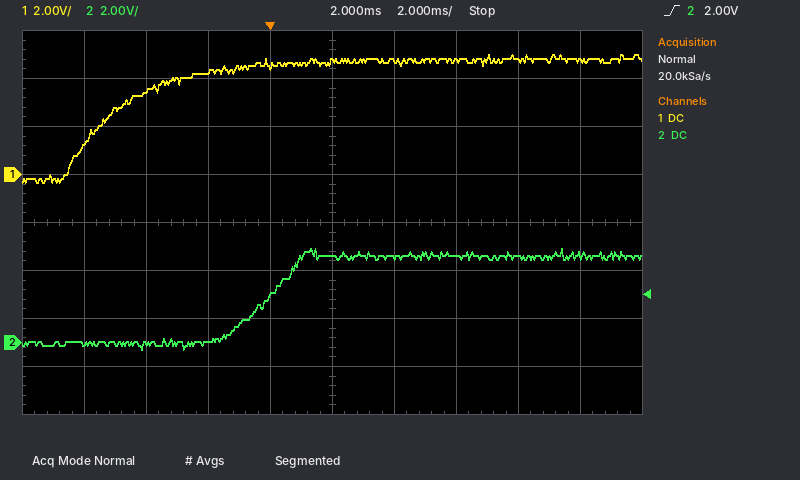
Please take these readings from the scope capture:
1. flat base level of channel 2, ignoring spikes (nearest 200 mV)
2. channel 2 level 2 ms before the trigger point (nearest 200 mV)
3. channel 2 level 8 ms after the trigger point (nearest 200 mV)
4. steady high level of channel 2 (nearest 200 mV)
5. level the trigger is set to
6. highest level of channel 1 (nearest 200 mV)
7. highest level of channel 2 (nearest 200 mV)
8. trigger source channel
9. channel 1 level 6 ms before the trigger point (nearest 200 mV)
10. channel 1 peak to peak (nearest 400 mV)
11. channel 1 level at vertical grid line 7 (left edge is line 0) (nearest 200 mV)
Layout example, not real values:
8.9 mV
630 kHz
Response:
0.0 V
0.0 V
3.6 V
3.6 V
2.00 V
5.0 V
4.0 V
channel 2
1.2 V
5.2 V
4.8 V
